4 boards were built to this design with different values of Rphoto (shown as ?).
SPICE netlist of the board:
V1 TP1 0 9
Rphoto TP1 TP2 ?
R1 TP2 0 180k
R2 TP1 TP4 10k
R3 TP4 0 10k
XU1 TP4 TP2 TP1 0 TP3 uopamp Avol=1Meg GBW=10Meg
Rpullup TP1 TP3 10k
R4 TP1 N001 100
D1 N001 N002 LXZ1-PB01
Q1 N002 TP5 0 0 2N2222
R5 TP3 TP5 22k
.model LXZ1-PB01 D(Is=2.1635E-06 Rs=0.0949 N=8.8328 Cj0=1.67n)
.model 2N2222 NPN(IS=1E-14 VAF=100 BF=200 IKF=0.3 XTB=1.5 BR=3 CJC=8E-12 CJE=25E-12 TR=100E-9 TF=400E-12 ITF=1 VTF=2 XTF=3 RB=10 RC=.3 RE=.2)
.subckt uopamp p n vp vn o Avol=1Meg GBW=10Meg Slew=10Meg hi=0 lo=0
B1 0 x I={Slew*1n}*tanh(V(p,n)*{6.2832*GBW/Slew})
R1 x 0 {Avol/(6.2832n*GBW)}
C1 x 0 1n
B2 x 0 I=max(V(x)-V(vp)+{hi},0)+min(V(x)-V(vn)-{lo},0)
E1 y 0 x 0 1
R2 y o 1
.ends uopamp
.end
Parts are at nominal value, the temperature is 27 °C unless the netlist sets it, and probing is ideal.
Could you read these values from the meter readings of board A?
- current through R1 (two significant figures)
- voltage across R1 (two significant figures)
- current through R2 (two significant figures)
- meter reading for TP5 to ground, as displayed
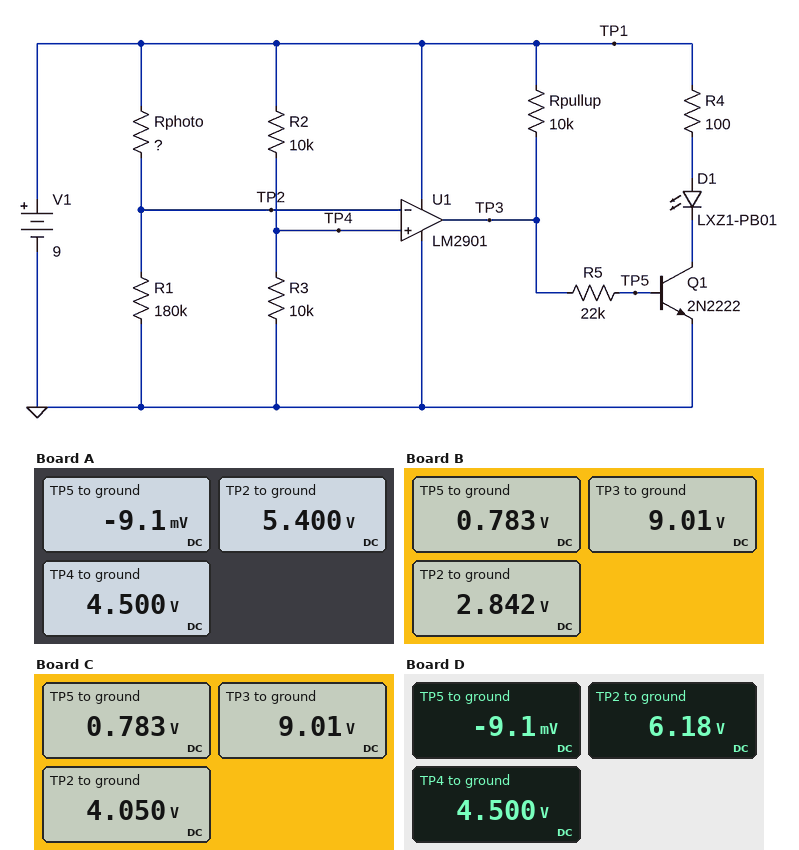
30 µA
5.4 V
450 µA
-9.1 mV
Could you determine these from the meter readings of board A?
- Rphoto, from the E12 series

120 kΩ
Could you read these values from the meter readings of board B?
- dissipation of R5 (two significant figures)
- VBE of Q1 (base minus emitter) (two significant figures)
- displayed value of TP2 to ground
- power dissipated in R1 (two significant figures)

3.1 mW
780 mV
2.842 V
45 µW
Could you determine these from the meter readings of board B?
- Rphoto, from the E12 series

390 kΩ
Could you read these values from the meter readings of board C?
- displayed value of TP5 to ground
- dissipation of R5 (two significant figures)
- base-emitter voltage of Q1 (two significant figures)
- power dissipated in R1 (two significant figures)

0.783 V
3.1 mW
780 mV
91 µW
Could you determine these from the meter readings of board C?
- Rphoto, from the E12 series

220 kΩ
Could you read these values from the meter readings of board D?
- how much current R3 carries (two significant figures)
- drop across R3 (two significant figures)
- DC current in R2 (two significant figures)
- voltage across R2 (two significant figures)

450 µA
4.5 V
450 µA
4.5 V
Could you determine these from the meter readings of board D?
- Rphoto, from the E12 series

82 kΩ
